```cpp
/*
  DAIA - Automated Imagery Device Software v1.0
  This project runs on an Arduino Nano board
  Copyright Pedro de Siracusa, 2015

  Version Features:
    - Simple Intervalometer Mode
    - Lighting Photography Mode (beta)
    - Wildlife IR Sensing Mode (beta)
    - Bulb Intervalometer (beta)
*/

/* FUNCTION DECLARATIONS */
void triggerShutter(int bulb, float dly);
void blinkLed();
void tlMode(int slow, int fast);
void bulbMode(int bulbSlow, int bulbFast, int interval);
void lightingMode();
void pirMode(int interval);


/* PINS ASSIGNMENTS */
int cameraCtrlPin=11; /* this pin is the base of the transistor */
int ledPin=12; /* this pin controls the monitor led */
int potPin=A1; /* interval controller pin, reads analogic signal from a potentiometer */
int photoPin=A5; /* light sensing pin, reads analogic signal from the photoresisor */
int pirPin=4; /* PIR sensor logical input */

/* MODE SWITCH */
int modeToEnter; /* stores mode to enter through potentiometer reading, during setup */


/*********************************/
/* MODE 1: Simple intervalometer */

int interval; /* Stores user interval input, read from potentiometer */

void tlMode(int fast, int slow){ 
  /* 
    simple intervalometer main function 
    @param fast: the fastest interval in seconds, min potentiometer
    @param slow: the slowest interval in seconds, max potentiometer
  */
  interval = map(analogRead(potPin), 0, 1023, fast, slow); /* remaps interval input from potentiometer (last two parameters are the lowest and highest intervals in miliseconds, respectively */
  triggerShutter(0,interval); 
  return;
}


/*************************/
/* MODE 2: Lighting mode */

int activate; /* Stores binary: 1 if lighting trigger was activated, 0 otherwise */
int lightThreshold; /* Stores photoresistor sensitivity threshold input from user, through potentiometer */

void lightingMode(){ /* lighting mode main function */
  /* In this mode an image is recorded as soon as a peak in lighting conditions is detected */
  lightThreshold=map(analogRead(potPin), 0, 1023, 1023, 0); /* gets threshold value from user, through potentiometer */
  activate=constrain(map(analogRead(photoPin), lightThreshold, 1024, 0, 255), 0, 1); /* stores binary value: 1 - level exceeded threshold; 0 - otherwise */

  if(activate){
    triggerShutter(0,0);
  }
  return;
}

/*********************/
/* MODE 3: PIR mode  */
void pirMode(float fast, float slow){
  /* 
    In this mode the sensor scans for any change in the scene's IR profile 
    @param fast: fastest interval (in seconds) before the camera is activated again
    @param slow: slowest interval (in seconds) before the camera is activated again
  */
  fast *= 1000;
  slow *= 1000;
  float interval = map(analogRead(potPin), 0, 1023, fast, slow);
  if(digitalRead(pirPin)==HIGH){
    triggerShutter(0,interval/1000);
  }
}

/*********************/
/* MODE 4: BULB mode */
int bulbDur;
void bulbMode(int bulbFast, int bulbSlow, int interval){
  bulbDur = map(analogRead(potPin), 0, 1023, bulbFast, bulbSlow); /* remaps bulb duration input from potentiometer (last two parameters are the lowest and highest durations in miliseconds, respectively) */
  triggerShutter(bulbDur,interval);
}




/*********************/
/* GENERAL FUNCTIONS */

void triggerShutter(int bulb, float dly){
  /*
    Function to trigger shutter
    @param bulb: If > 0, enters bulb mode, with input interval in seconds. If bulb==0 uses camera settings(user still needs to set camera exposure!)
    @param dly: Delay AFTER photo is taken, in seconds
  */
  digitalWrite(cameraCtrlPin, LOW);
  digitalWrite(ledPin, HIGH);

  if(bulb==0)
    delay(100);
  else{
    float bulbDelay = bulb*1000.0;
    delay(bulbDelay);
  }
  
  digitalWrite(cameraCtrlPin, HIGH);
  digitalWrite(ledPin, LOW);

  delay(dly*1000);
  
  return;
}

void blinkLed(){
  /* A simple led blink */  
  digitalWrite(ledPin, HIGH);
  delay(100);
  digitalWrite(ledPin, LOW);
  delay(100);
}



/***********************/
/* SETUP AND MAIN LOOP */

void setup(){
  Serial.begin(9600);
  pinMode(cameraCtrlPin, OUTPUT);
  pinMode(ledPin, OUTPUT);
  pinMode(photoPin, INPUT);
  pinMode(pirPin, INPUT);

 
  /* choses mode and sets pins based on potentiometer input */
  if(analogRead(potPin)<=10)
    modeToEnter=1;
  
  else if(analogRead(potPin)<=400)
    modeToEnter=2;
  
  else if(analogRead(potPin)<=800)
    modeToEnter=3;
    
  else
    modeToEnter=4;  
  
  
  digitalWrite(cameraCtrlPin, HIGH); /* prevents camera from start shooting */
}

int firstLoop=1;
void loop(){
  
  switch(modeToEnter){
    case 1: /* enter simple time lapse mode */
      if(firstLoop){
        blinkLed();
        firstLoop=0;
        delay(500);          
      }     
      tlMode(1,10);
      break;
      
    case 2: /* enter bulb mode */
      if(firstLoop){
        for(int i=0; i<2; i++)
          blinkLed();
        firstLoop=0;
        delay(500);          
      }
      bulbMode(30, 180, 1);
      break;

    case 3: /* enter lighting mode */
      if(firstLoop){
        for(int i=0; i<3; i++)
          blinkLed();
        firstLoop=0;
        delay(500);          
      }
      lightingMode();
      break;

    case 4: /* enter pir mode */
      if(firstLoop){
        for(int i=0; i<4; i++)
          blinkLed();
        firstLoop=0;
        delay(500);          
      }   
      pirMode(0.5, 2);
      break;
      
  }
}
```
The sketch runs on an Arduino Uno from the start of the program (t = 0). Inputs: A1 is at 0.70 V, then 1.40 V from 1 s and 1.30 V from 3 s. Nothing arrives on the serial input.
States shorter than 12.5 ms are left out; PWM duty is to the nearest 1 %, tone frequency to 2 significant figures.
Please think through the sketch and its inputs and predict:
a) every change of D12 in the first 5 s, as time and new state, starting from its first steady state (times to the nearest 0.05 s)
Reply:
0 s high; 0.1 s low; 0.2 s high; 0.3 s low; 0.9 s high
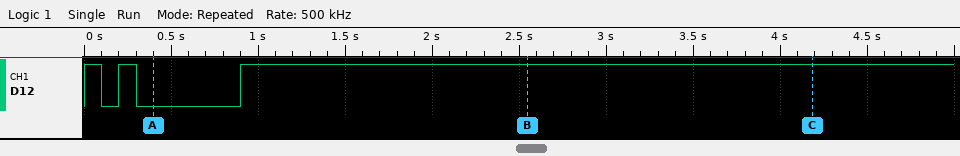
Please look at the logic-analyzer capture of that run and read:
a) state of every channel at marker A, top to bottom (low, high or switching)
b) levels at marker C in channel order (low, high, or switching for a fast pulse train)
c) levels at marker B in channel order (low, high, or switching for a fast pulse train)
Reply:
D12 low
D12 high
D12 high
